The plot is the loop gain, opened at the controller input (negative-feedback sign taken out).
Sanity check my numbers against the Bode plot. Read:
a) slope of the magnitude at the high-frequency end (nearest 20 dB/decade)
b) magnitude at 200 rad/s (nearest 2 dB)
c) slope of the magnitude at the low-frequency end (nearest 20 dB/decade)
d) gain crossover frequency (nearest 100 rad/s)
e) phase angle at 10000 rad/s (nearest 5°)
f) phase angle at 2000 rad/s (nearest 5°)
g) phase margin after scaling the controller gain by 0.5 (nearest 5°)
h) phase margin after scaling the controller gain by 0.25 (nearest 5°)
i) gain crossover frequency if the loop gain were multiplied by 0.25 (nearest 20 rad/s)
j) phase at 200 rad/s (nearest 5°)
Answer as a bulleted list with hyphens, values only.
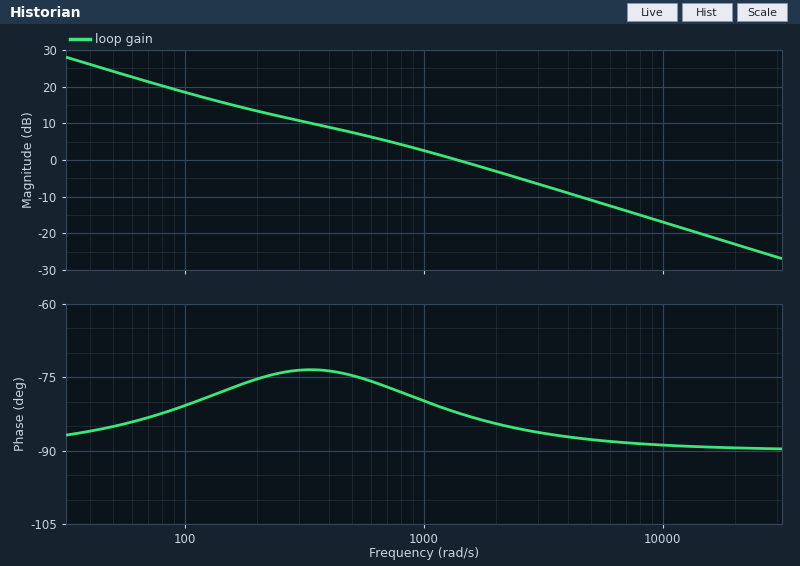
- -20 dB/decade
- 14 dB
- -20 dB/decade
- 1400 rad/s
- -90°
- -85°
- 105°
- 105°
- 240 rad/s
- -75°
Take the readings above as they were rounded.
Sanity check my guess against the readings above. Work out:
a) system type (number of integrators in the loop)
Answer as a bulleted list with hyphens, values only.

- 1
